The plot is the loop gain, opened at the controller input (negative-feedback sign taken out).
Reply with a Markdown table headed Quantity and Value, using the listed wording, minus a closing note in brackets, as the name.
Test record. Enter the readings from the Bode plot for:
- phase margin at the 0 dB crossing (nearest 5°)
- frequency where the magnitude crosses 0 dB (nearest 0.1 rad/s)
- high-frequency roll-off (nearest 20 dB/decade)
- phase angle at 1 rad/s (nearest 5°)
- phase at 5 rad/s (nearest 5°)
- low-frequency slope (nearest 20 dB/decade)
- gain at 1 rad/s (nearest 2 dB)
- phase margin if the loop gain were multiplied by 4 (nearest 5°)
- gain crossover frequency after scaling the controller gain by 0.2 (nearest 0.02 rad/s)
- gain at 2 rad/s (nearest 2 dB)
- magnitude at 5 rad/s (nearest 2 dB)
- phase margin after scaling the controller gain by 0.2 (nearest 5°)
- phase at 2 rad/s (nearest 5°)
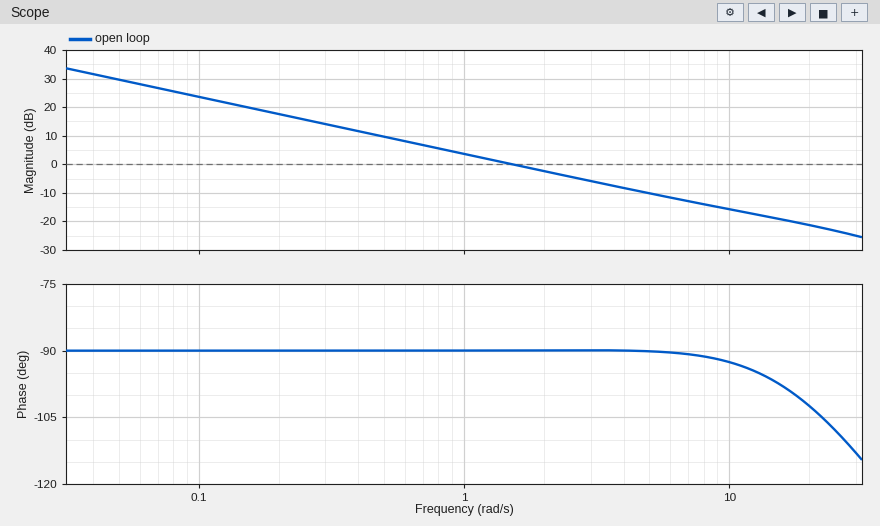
| Quantity | Value |
|---|---|
| phase margin at the 0 dB crossing | 90° |
| frequency where the magnitude crosses 0 dB | 1.5 rad/s |
| high-frequency roll-off | -20 dB/decade |
| phase angle at 1 rad/s | -90° |
| phase at 5 rad/s | -90° |
| low-frequency slope | -20 dB/decade |
| gain at 1 rad/s | 4 dB |
| phase margin if the loop gain were multiplied by 4 | 90° |
| gain crossover frequency after scaling the controller gain by 0.2 | 0.30 rad/s |
| gain at 2 rad/s | -2 dB |
| magnitude at 5 rad/s | -10 dB |
| phase margin after scaling the controller gain by 0.2 | 90° |
| phase at 2 rad/s | -90° |
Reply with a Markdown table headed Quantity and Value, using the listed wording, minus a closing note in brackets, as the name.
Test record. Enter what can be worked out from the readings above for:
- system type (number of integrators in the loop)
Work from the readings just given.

| Quantity | Value |
|---|---|
| system type | 1 |
